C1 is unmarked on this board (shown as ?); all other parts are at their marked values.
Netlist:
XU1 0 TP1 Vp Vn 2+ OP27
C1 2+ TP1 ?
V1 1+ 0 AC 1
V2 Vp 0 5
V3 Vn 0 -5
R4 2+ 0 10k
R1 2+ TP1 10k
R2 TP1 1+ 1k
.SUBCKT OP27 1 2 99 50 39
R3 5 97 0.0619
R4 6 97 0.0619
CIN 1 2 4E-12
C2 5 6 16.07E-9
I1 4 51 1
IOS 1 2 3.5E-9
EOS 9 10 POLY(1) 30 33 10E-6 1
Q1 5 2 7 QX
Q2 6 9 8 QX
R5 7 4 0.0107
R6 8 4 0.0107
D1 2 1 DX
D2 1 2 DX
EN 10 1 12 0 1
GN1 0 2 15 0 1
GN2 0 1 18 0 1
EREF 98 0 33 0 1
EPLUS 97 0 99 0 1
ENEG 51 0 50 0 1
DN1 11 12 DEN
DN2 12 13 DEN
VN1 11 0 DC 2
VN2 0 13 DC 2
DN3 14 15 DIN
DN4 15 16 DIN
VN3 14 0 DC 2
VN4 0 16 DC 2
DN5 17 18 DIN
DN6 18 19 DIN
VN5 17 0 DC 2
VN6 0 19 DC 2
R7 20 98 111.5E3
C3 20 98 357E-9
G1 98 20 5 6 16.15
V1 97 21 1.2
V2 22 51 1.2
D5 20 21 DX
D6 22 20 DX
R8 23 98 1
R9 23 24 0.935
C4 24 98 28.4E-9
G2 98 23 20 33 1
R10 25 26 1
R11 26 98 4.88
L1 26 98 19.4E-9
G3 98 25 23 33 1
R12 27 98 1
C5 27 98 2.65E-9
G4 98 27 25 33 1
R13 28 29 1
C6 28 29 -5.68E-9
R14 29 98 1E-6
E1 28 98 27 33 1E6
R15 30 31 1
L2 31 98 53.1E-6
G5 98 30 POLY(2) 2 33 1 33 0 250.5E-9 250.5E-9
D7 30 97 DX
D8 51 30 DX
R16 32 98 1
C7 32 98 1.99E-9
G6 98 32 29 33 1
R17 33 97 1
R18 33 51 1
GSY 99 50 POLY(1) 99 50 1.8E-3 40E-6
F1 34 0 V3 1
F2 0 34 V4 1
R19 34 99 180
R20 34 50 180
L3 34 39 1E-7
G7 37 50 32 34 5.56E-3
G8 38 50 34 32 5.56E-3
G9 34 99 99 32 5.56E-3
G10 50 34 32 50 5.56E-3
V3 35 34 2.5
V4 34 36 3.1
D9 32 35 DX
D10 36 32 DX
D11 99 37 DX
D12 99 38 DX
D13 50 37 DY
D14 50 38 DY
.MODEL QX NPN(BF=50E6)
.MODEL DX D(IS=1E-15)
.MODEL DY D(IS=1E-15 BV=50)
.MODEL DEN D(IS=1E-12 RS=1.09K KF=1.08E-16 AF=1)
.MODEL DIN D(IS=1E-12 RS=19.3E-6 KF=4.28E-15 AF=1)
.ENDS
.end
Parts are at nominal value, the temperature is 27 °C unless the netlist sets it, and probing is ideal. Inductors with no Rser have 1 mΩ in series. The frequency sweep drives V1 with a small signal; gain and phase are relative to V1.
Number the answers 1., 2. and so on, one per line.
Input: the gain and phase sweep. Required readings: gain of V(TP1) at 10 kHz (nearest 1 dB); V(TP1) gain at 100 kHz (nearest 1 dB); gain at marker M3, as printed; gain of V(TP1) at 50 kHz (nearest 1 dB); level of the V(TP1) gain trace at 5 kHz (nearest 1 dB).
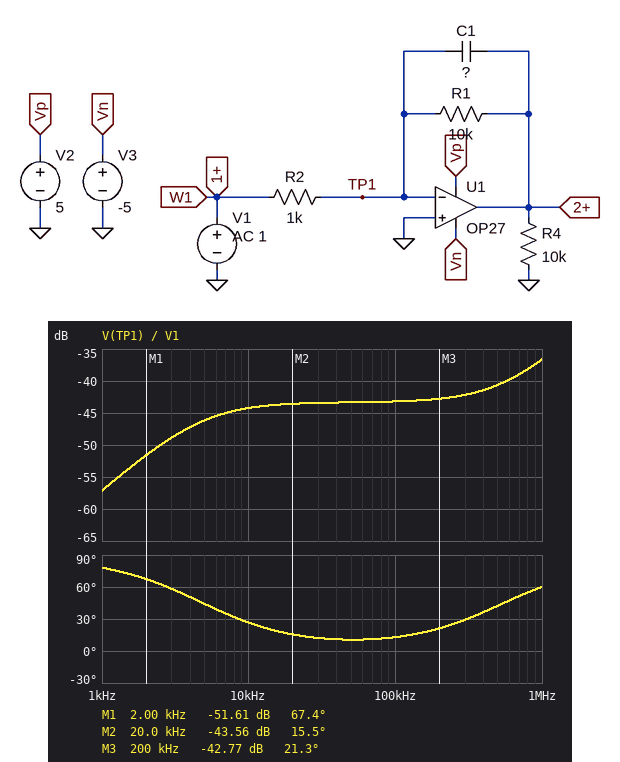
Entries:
1. -44 dB
2. -43 dB
3. -42.77 dB
4. -43 dB
5. -46 dB
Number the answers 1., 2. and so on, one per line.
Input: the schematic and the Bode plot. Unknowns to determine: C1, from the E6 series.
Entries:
1. 3.3 nF
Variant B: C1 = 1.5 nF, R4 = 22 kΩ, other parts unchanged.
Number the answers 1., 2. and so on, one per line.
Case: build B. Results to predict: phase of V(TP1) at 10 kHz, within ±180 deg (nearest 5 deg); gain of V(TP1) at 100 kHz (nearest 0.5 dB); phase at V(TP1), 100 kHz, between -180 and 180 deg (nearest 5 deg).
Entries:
1. 45 deg
2. -36.5 dB
3. 10 deg
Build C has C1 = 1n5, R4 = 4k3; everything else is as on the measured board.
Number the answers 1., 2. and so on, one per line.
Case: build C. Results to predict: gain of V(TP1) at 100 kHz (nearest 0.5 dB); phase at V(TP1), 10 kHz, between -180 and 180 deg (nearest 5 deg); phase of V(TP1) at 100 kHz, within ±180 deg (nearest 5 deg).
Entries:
1. -36.5 dB
2. 45 deg
3. 10 deg
